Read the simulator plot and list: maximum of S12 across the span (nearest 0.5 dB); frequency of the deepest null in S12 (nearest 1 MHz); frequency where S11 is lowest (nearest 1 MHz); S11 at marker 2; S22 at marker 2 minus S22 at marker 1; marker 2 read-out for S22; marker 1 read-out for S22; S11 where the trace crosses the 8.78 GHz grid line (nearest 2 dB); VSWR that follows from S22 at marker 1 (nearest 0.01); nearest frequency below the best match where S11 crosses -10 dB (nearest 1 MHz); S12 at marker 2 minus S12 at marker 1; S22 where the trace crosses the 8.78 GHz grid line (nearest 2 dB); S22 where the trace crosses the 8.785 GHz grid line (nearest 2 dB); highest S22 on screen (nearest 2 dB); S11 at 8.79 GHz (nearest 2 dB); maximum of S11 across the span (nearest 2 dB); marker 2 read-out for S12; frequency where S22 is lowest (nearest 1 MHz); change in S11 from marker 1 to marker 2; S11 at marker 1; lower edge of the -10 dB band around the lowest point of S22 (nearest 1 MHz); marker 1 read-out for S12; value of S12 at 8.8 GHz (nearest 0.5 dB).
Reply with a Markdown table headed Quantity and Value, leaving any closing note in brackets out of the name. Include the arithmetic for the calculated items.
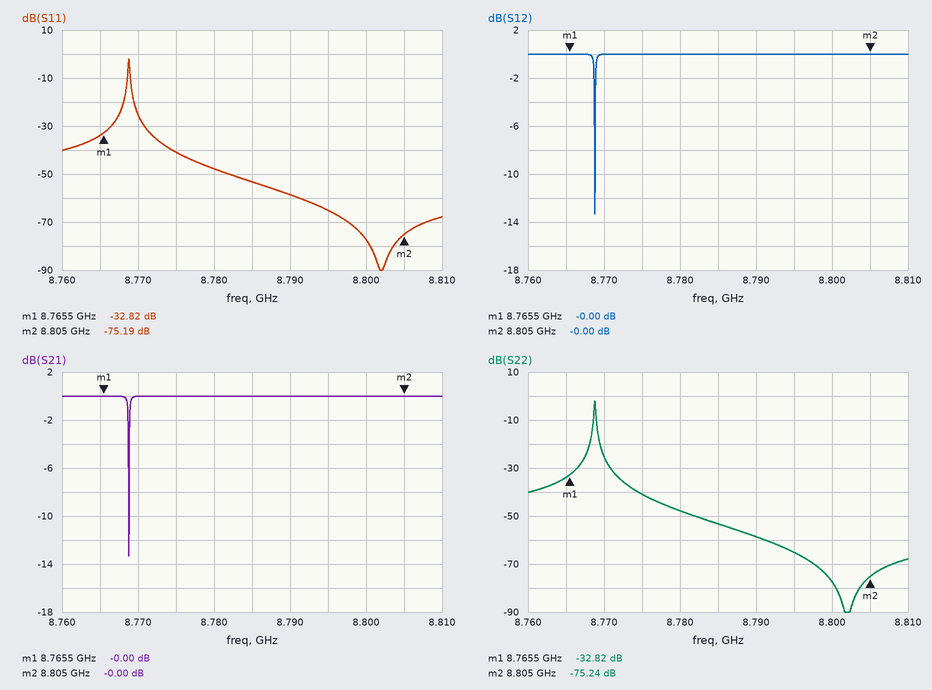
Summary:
| Quantity | Value |
|---|---|
| maximum of S12 across the span | 0.0 dB |
| frequency of the deepest null in S12 | 8.769 GHz |
| frequency where S11 is lowest | 8.802 GHz |
| S11 at marker 2 | -75.19 dB |
| S22 at marker 2 minus S22 at marker 1 | -75.24 − (-32.82) = -42.42 dB |
| marker 2 read-out for S22 | -75.24 dB |
| marker 1 read-out for S22 | -32.82 dB |
| S11 where the trace crosses the 8.78 GHz grid line | -48 dB |
| VSWR that follows from S22 at marker 1 | (1 + 0.0229)/(1 − 0.0229) ≈ 1.05 |
| nearest frequency below the best match where S11 crosses -10 dB | 8.769 GHz |
| S12 at marker 2 minus S12 at marker 1 | -0 − (-0) = 0.00 dB |
| S22 where the trace crosses the 8.78 GHz grid line | -48 dB |
| S22 where the trace crosses the 8.785 GHz grid line | -54 dB |
| highest S22 on screen | -2 dB |
| S11 at 8.79 GHz | -58 dB |
| maximum of S11 across the span | -2 dB |
| marker 2 read-out for S12 | -0.00 dB |
| frequency where S22 is lowest | 8.802 GHz |
| change in S11 from marker 1 to marker 2 | -75.19 − (-32.82) = -42.37 dB |
| S11 at marker 1 | -32.82 dB |
| lower edge of the -10 dB band around the lowest point of S22 | 8.769 GHz |
| marker 1 read-out for S12 | -0.00 dB |
| value of S12 at 8.8 GHz | 0.0 dB |
